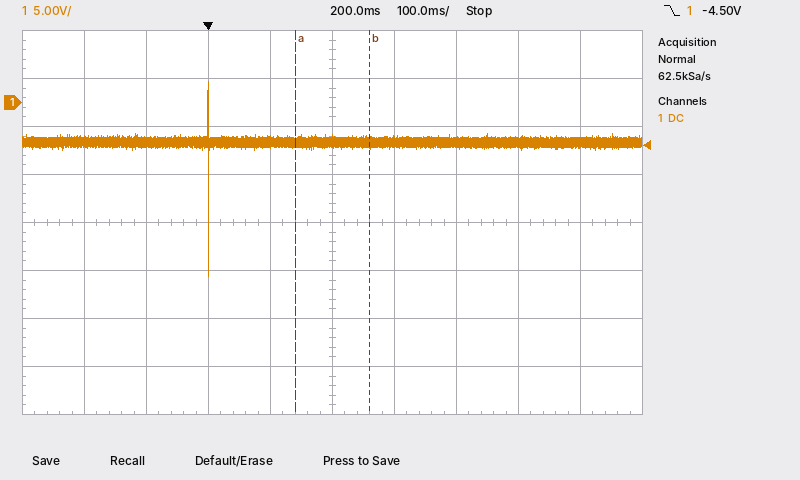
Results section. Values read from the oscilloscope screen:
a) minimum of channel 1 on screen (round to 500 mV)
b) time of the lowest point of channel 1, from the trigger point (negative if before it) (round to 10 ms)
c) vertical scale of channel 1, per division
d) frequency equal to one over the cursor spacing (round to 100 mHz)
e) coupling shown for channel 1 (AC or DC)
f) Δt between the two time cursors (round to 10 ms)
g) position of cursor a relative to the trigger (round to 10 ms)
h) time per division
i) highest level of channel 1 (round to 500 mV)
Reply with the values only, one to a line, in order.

-18.0 V
0 ms
5 V
8.3 Hz
DC
120 ms
+140 ms
100 ms
2.0 V
